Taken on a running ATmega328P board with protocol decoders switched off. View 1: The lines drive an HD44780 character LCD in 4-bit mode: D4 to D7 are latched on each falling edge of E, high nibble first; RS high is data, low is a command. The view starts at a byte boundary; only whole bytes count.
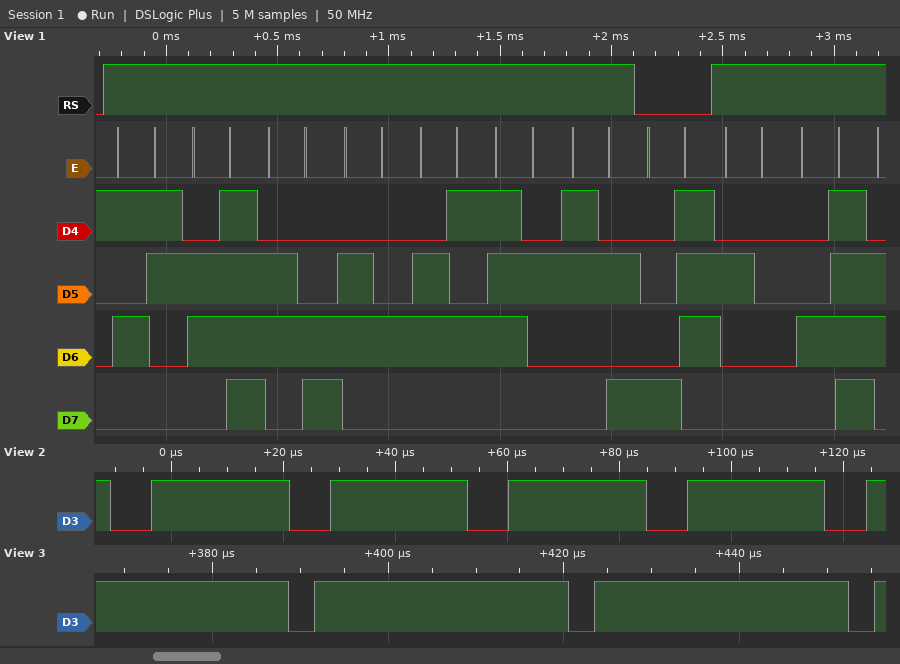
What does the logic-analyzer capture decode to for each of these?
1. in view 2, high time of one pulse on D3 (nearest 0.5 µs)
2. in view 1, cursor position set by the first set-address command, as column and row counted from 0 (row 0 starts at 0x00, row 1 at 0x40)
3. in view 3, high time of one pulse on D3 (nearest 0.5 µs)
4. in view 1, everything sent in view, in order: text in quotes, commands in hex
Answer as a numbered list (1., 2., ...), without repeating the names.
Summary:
1. 24.5 µs
2. column 7, row 0
3. 29.0 µs
4. "Solder:" 0x87 " O"
